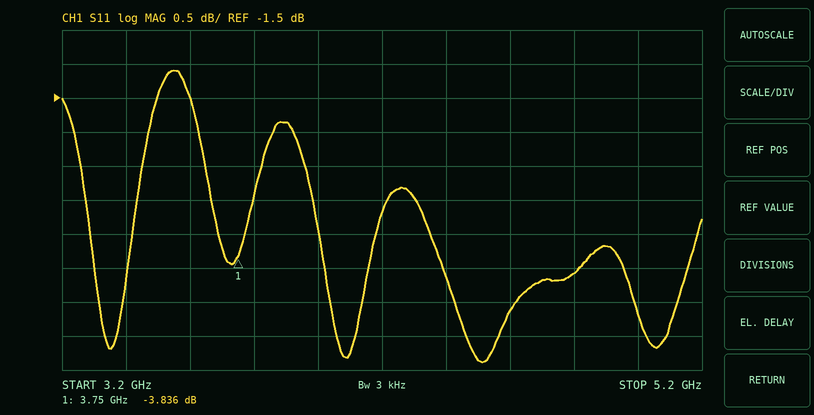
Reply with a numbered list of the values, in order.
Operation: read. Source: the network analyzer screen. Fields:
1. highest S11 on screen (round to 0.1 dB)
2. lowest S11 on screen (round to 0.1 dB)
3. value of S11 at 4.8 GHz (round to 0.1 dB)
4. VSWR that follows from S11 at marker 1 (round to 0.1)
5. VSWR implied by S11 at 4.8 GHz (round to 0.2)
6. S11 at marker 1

1. -1.1 dB
2. -5.4 dB
3. -4.1 dB
4. 4.6
5. 4.4
6. -3.836 dB
